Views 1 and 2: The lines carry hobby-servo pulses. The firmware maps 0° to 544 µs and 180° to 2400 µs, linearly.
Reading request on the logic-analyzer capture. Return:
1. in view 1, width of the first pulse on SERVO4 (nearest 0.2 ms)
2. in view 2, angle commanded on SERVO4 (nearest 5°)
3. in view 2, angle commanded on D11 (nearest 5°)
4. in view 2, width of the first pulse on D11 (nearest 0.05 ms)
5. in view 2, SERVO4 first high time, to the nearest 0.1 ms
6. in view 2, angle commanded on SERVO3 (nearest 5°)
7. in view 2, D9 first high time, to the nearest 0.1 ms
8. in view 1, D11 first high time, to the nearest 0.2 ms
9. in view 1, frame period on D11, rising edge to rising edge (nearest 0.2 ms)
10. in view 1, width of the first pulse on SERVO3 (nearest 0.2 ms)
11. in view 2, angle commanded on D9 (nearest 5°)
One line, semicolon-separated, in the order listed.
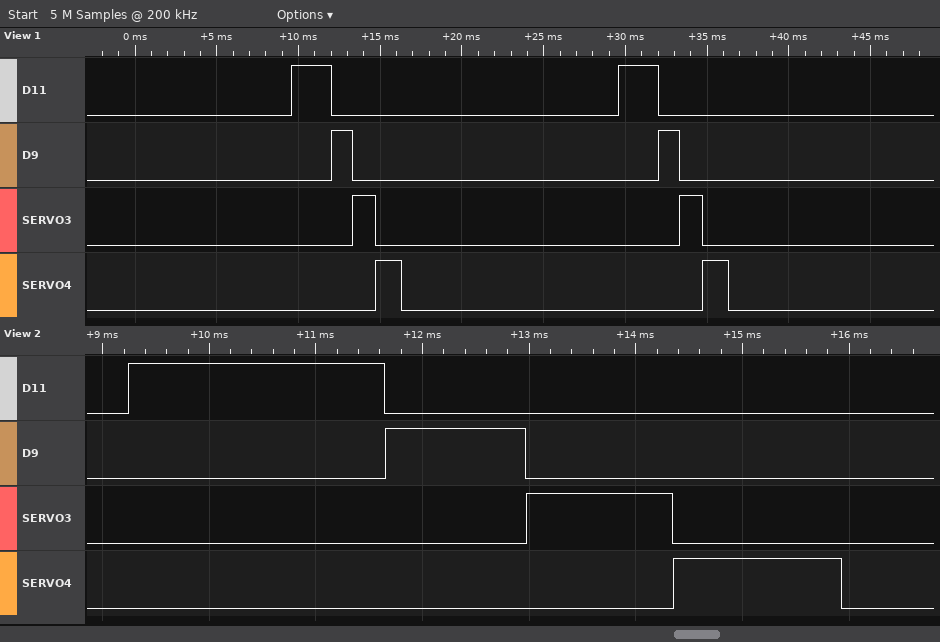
1.6 ms; 100°; 180°; 2.40 ms; 1.6 ms; 80°; 1.3 ms; 2.4 ms; 20.0 ms; 1.4 ms; 75°
